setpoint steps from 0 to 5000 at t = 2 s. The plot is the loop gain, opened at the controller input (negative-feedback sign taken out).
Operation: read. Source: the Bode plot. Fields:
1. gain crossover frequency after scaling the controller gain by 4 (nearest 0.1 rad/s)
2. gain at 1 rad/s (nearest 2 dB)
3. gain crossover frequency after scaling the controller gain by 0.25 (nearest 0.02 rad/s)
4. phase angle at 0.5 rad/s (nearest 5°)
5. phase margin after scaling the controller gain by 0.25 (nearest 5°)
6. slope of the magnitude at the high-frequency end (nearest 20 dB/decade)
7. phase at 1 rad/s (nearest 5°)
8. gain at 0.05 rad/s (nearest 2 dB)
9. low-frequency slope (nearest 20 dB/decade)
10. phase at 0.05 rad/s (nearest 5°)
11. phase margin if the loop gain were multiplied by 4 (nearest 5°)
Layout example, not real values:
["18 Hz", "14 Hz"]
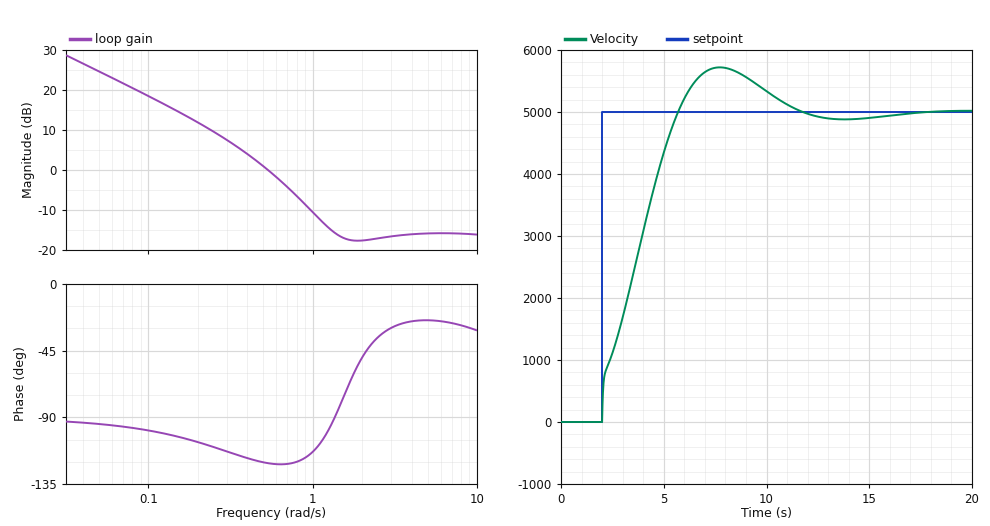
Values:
["1.1 rad/s", "-10 dB", "0.20 rad/s", "-120°", "75°", "0 dB/decade", "-115°", "24 dB", "-20 dB/decade", "-95°", "70°"]
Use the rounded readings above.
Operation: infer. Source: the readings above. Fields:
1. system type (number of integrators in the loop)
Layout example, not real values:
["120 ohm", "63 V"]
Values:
["1"]
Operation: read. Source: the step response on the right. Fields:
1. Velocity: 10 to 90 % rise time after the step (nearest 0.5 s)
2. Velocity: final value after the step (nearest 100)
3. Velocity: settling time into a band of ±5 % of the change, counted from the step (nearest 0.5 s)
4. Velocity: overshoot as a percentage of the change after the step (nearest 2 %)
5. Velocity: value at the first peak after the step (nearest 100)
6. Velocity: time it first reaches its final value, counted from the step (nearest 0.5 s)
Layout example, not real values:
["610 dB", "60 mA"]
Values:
["3.0 s", "5000", "8.5 s", "14 %", "5700", "3.5 s"]
